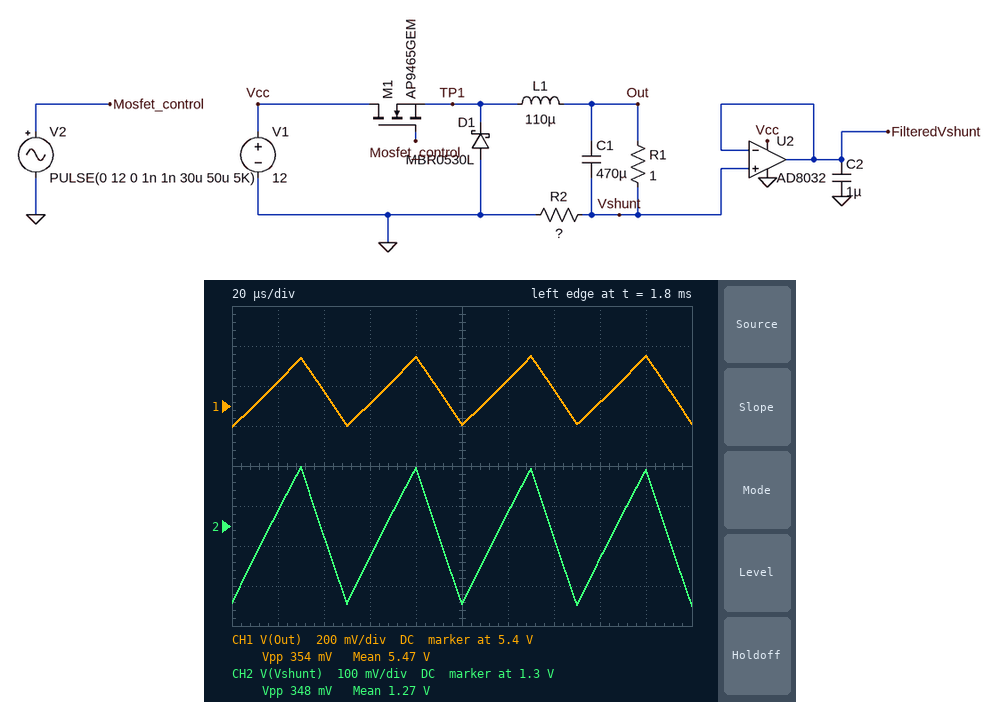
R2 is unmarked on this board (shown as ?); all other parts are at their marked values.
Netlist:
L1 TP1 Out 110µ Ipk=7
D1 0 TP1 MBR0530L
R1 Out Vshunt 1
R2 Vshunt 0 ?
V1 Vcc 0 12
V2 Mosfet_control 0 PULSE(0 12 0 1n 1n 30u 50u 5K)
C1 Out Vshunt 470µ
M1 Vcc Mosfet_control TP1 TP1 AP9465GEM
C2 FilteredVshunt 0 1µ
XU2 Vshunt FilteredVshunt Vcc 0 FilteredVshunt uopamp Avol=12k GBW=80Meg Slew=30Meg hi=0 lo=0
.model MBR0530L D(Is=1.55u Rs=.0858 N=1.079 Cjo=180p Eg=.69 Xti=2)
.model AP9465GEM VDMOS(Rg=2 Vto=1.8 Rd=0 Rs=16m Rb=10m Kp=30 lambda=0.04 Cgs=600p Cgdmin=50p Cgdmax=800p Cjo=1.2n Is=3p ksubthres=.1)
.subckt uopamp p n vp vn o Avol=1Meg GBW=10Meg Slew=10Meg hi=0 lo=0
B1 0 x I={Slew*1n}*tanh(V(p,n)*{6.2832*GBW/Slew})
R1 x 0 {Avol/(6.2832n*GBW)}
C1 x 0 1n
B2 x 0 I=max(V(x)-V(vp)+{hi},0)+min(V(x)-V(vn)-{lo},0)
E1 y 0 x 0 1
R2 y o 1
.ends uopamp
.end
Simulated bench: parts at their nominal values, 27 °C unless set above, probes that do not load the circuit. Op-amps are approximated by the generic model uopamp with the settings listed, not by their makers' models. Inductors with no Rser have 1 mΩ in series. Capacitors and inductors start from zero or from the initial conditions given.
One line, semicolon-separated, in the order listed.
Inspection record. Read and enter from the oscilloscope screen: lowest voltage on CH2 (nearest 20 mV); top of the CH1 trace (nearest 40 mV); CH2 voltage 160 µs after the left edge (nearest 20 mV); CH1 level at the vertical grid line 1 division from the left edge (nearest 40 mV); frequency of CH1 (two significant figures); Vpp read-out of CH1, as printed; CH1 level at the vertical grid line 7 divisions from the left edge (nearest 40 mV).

1.10 V; 5.64 V; 1.22 V; 5.52 V; 20 kHz; 354 mV; 5.48 V
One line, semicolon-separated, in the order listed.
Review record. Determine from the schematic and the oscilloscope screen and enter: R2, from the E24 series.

0.3 Ω
